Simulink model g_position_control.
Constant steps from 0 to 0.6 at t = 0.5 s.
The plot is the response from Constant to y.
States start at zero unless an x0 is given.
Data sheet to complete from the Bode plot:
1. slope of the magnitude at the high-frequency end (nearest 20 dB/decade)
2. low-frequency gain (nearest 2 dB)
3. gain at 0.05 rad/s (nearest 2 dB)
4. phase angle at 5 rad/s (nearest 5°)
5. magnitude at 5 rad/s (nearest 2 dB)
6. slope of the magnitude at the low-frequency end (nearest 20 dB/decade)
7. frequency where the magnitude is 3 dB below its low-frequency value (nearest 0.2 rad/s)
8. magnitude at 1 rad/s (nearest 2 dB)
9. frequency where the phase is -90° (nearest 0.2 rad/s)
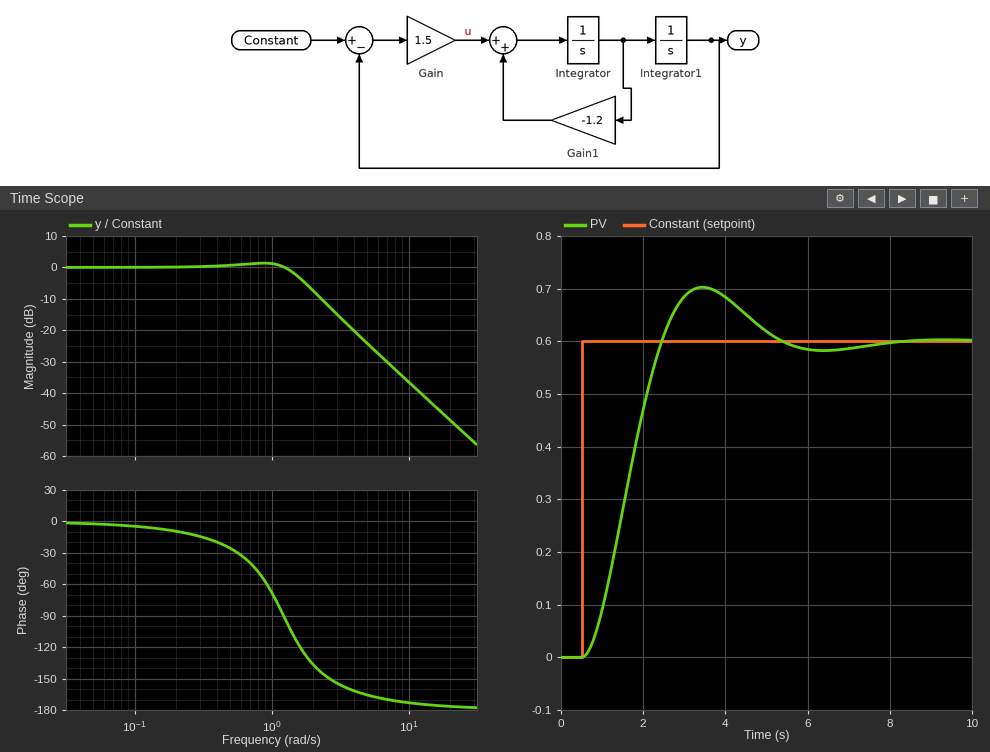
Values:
-40 dB/decade
0 dB
0 dB
-165°
-24 dB
0 dB/decade
1.6 rad/s
2 dB
1.2 rad/s
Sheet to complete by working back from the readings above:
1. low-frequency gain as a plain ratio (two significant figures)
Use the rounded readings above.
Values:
1.0
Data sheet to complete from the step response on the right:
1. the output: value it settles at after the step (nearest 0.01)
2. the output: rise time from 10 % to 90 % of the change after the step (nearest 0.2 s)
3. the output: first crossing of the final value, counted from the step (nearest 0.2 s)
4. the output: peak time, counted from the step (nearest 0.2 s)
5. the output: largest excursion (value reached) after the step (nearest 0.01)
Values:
0.60
1.4 s
2.0 s
3.0 s
0.70
